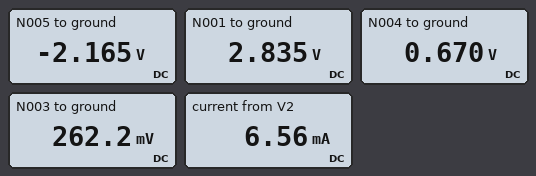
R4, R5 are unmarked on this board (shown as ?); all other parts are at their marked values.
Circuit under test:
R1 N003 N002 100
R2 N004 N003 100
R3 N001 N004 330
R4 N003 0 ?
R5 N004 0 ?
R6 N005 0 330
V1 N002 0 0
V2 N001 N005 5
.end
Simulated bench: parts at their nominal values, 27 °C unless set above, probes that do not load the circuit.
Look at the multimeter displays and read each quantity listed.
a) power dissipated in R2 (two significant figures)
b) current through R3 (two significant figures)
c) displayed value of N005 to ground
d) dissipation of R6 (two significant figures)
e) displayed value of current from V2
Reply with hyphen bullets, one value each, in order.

- 1.7 mW
- 6.6 mA
- -2.165 V
- 14 mW
- 6.56 mA
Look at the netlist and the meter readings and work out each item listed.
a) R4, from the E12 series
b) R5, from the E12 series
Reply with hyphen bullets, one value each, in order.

- 180 Ω
- 270 Ω
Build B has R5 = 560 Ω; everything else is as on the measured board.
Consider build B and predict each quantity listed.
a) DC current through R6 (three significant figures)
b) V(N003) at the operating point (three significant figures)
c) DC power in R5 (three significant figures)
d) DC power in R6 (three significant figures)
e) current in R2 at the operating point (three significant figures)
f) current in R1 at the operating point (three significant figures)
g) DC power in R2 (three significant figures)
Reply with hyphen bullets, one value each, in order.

- 6.35 mA
- 316 mV
- 1.16 mW
- 13.3 mW
- 4.91 mA
- 3.16 mA
- 2.41 mW
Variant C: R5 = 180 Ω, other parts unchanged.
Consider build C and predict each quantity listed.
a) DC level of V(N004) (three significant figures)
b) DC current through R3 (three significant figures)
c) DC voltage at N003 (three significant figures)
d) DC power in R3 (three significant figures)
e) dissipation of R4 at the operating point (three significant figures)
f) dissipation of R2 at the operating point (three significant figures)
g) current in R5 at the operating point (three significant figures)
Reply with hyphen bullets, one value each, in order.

- 576 mV
- 6.70 mA
- 225 mV
- 14.8 mW
- 282 µW
- 1.23 mW
- 3.20 mA
